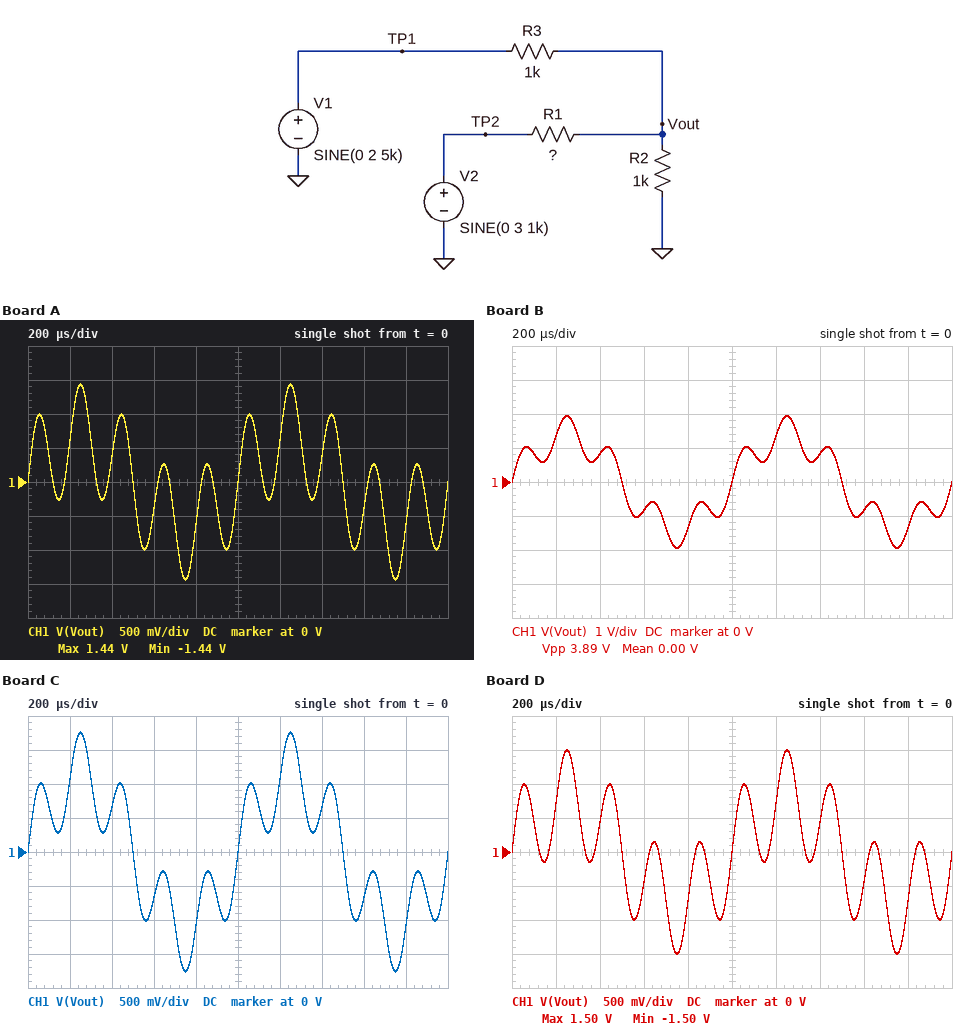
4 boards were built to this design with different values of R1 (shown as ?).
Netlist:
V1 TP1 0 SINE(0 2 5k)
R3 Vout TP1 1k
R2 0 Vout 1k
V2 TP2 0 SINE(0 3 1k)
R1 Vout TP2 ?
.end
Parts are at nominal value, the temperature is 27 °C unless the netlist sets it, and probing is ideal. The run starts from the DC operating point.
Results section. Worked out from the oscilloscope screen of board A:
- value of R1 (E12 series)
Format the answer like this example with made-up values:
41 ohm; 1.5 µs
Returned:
1.8 kΩ
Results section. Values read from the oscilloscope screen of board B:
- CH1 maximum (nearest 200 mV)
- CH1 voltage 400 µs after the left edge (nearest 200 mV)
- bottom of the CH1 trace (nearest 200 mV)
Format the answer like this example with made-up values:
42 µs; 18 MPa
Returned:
2.0 V; 800 mV; -2.0 V
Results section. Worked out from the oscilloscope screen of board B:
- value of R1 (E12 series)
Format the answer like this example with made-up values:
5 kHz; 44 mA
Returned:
560 Ω
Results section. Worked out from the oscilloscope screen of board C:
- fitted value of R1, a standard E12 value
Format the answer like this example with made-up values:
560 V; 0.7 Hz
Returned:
820 Ω
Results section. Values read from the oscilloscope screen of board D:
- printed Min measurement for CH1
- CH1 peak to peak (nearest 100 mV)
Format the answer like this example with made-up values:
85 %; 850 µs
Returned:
-1.50 V; 3.0 V
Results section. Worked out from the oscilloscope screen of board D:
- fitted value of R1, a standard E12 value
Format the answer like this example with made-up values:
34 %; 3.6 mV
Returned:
1.5 kΩ
